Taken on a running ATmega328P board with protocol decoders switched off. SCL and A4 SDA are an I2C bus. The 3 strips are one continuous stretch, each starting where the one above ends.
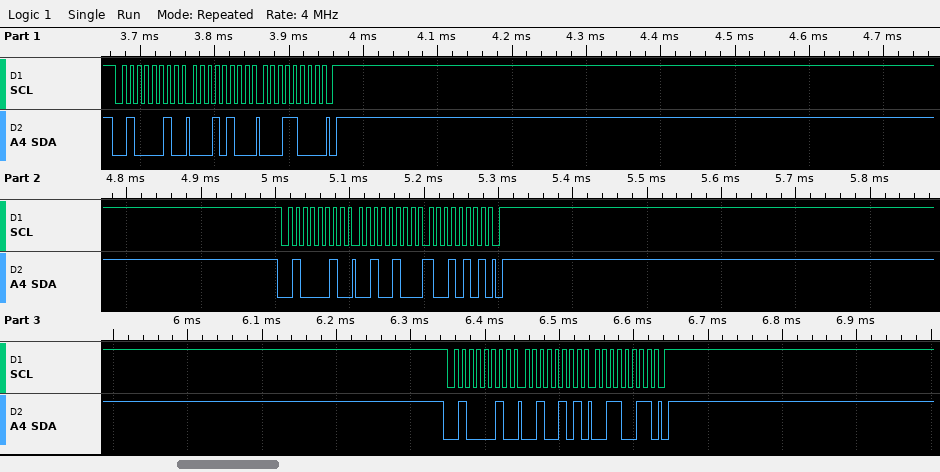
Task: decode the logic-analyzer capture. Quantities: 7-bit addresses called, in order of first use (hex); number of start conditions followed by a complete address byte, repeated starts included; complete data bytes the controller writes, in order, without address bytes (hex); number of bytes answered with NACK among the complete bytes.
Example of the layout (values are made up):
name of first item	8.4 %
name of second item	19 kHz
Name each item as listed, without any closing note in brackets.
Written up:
7-bit addresses called, in order of first use	0x21
number of start conditions followed by a complete address byte, repeated starts included	3
complete data bytes the controller writes, in order, without address bytes	14 18 24 95 25 33
number of bytes answered with NACK among the complete bytes	0
